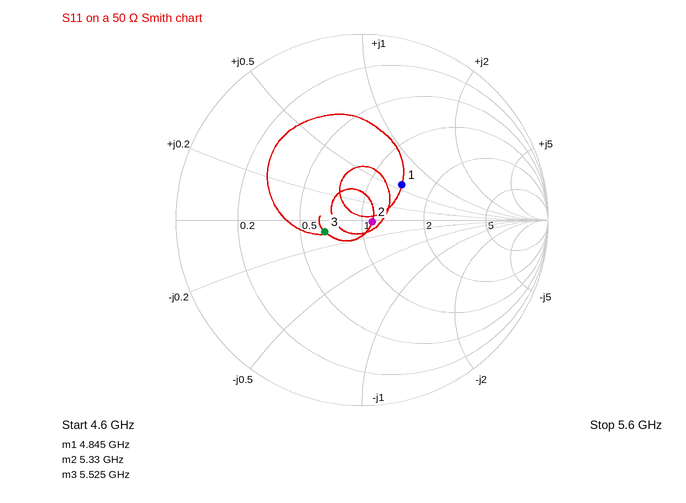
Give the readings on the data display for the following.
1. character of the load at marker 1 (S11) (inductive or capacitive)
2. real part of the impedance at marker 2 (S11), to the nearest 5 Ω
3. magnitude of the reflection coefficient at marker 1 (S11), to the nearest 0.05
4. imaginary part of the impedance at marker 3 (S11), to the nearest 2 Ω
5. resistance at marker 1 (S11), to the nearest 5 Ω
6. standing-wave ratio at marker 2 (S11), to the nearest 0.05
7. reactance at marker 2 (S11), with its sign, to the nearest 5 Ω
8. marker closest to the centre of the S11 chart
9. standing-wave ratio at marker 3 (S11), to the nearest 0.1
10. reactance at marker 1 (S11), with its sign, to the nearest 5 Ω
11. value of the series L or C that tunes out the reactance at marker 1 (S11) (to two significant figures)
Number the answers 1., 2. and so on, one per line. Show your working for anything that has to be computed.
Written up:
1. inductive
2. 55 Ω
3. 0.30
4. -4 Ω
5. 70 Ω
6. 1.10
7. 0 Ω
8. marker 2
9. 1.5
10. +30 Ω
11. C = 1/(2π × 4.845 GHz × 30 Ω) ≈ 1.1 pF
